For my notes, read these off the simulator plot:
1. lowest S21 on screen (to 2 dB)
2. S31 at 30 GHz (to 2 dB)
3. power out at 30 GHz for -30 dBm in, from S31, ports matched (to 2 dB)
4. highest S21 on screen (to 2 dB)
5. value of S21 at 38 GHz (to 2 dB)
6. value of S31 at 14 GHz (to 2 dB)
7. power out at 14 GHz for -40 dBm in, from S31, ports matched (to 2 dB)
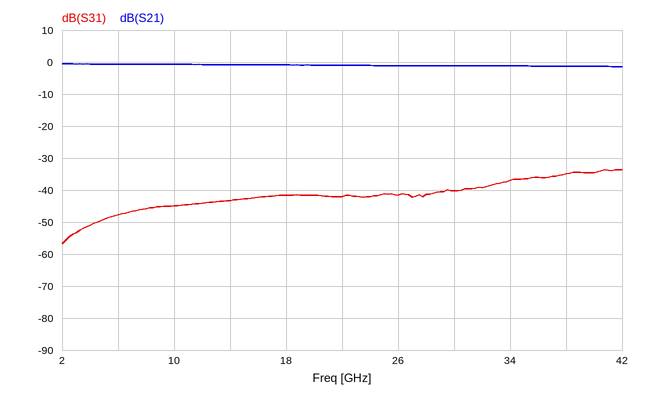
-2 dB
-40 dB
-70 dBm
0 dB
-2 dB
-44 dB
-84 dBm
